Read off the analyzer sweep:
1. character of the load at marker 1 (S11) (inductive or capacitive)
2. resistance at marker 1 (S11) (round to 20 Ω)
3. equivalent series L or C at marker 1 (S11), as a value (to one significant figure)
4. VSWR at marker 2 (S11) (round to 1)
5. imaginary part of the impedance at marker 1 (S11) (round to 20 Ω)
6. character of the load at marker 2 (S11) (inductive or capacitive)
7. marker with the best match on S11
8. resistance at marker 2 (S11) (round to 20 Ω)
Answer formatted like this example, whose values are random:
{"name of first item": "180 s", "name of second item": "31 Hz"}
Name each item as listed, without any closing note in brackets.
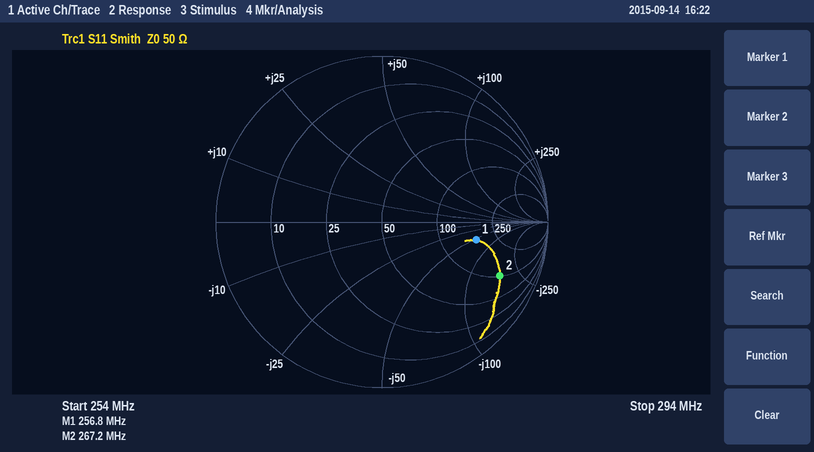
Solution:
{"character of the load at marker 1 (S11)": "capacitive", "resistance at marker 1 (S11)": "160 Ω", "equivalent series L or C at marker 1 (S11), as a value": "10 pF", "VSWR at marker 2 (S11)": "8", "imaginary part of the impedance at marker 1 (S11)": "-60 Ω", "character of the load at marker 2 (S11)": "capacitive", "marker with the best match on S11": "marker 1", "resistance at marker 2 (S11)": "100 Ω"}
